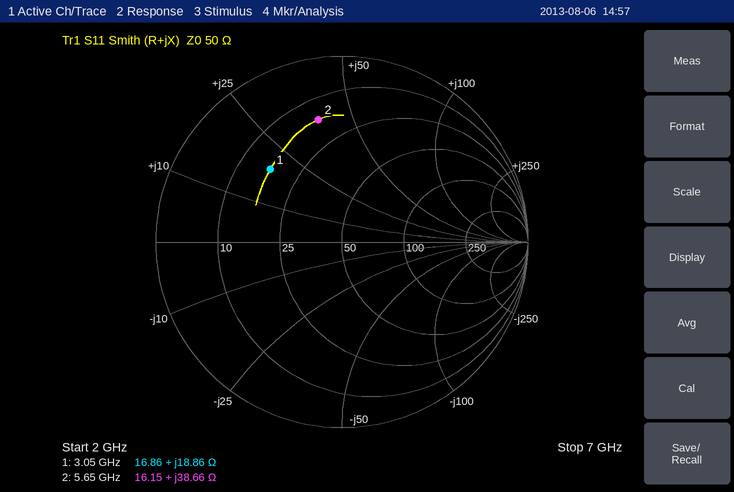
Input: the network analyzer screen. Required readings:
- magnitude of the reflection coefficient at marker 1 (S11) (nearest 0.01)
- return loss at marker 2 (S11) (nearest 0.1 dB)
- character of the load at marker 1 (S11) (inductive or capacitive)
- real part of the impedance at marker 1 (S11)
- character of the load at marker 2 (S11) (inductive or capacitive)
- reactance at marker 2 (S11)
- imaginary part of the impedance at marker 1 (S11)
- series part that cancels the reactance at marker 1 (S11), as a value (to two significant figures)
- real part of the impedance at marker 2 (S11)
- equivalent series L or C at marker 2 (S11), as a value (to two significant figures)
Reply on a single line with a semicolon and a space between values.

0.55; 3.5 dB; inductive; 16.86 Ω; inductive; +38.66 Ω; +18.86 Ω; 2.8 pF; 16.15 Ω; 1.1 nH
